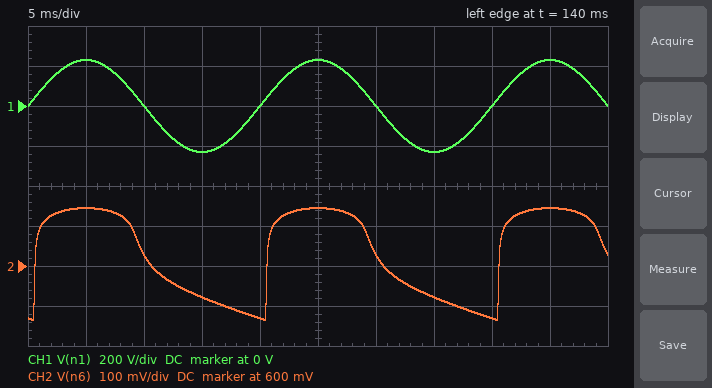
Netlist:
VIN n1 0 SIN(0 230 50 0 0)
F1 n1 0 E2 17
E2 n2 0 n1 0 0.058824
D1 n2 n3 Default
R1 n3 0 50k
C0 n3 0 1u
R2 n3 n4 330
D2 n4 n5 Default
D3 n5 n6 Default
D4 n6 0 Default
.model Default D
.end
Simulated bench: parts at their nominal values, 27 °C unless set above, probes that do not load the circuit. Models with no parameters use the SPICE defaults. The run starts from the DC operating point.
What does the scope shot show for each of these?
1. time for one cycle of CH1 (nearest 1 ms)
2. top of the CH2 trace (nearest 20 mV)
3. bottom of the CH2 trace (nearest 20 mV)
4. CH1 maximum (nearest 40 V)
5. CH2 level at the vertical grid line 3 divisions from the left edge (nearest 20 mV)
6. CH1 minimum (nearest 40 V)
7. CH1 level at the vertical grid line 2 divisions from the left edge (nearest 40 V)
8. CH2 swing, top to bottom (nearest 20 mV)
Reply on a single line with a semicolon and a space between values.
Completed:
20 ms; 740 mV; 460 mV; 240 V; 520 mV; -240 V; 0 V; 280 mV
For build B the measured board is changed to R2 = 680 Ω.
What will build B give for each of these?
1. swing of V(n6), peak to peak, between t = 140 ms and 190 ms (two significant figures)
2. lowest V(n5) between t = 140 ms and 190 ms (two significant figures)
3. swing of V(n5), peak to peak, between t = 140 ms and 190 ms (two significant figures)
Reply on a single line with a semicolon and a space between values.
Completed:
250 mV; 950 mV; 500 mV
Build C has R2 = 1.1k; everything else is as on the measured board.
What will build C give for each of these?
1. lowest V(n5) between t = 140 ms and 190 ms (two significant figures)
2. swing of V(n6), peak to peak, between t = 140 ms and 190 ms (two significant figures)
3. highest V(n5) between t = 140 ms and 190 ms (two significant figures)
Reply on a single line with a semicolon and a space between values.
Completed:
980 mV; 220 mV; 1.4 V
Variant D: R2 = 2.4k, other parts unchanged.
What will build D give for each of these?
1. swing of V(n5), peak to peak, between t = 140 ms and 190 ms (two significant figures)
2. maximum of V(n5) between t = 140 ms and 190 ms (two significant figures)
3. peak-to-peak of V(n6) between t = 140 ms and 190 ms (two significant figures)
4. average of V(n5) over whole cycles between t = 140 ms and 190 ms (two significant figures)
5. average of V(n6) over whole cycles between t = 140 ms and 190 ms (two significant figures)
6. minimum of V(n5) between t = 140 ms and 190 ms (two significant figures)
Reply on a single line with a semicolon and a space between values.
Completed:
320 mV; 1.4 V; 160 mV; 1.3 V; 630 mV; 1.1 V
